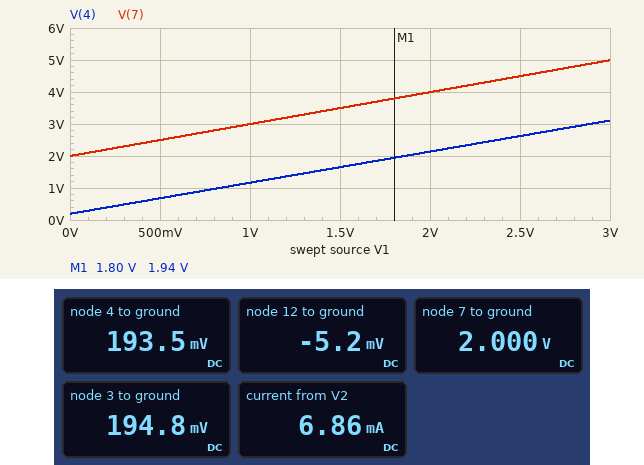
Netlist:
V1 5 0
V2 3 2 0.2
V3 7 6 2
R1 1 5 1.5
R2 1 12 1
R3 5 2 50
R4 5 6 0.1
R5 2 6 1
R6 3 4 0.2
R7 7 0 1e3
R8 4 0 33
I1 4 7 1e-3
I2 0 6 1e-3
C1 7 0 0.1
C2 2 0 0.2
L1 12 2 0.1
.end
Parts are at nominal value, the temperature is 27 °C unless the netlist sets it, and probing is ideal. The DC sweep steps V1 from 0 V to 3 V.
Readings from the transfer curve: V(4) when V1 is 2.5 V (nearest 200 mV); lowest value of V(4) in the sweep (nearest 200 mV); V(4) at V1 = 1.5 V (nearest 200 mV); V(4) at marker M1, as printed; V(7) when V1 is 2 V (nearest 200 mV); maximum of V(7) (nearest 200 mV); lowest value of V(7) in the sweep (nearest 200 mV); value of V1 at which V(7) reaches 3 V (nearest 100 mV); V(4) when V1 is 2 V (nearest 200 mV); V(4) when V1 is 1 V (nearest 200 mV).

2.6 V
200 mV
1.6 V
1.94 V
4.0 V
5.0 V
2.0 V
1.0 V
2.2 V
1.2 V
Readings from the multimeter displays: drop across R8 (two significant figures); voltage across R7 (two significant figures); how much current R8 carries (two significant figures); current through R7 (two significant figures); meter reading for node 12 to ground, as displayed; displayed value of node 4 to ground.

190 mV
2.0 V
5.9 mA
2.0 mA
-5.2 mV
193.5 mV
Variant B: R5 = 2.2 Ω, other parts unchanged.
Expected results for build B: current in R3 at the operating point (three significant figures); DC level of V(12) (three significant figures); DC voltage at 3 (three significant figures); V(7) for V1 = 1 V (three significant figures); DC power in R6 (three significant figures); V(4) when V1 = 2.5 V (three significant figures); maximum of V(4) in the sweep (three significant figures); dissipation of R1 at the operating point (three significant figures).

159 µA
-7.93 mV
192 mV
3.00 V
9.19 µW
2.59 V
3.07 V
15.1 µW
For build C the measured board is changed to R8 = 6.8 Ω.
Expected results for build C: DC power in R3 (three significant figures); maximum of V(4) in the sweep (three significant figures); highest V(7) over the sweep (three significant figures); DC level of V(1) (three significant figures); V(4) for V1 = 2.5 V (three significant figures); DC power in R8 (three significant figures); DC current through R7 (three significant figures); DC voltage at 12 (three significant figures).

8.06 µW
2.81 V
4.97 V
-12.0 mV
2.37 V
4.48 mW
2.00 mA
-20.1 mV
